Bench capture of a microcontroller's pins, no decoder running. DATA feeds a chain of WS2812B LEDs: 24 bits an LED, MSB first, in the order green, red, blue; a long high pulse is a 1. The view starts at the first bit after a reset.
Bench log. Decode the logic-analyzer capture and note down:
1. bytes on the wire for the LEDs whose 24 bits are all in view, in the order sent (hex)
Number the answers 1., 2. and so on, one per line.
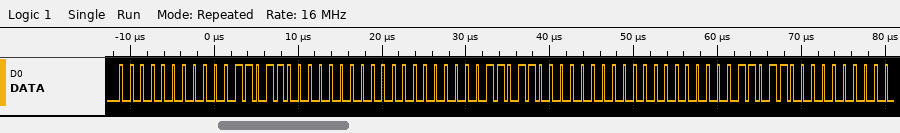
1. 00 1B 00 00 1B 00 00 1B 00
